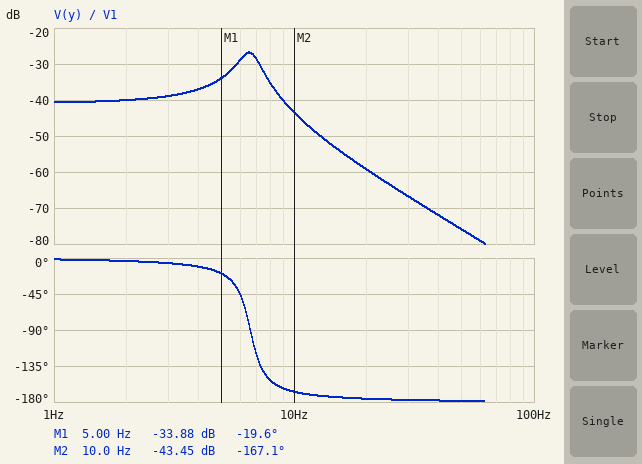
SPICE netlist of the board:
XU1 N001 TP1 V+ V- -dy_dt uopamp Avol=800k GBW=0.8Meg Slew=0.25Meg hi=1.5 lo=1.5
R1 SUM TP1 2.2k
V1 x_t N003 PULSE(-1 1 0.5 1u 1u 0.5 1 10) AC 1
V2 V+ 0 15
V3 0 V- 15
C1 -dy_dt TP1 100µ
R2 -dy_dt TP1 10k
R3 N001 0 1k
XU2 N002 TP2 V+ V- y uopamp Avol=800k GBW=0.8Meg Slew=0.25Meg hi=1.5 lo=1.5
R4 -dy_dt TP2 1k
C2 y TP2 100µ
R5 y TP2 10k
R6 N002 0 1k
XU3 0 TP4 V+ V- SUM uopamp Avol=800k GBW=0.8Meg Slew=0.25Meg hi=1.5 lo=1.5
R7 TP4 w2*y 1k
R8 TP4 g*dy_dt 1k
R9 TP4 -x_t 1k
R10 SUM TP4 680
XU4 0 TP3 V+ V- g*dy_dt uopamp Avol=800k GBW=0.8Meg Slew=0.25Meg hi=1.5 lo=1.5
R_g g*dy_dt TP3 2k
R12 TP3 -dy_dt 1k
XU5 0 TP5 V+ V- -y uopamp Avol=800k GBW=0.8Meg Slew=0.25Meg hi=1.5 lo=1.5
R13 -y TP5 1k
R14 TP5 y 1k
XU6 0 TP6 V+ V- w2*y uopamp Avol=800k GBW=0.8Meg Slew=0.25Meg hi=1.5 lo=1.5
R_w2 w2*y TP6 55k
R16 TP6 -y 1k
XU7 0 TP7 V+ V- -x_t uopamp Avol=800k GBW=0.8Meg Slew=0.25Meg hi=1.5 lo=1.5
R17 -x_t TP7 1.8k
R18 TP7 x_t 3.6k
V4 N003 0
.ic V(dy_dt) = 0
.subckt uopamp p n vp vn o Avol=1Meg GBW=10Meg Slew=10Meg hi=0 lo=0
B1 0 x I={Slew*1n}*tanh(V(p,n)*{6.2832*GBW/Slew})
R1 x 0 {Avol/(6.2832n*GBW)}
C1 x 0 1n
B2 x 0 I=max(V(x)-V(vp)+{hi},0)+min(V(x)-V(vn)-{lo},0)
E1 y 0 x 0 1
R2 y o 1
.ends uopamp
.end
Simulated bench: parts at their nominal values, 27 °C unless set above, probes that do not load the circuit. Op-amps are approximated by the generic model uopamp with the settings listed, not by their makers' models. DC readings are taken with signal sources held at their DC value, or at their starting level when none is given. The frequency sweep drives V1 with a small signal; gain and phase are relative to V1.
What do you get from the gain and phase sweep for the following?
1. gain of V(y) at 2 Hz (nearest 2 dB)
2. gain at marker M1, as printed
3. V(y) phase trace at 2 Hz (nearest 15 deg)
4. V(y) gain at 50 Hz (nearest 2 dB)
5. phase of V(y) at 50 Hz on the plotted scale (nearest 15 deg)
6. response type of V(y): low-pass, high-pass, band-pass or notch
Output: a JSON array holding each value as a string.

["-40 dB", "-33.88 dB", "0 deg", "-76 dB", "-180 deg", "low-pass"]
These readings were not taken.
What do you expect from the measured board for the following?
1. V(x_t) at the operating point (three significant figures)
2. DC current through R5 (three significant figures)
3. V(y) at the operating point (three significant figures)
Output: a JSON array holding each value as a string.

["-1.00 V", "905 nA", "-9.05 mV"]
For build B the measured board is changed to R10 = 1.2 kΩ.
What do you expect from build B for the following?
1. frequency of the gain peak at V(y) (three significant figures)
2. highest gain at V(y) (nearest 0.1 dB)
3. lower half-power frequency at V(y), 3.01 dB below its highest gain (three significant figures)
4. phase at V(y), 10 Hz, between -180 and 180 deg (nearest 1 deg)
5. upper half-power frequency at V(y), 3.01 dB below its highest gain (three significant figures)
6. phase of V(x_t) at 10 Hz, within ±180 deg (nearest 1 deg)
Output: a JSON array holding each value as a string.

["8.61 Hz", "-28.2 dB", "7.51 Hz", "-139 deg", "9.59 Hz", "0 deg"]
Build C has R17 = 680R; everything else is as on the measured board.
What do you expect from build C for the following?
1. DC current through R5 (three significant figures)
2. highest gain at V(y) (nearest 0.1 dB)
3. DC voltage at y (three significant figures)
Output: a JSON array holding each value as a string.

["342 nA", "-35.2 dB", "-3.42 mV"]
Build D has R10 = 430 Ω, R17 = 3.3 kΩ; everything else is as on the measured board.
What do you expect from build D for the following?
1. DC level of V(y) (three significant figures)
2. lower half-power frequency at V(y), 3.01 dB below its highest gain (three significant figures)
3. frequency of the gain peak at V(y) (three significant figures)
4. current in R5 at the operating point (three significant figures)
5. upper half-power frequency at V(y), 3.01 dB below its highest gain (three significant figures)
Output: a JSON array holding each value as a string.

["-16.6 mV", "4.69 Hz", "5.19 Hz", "1.66 µA", "5.64 Hz"]
